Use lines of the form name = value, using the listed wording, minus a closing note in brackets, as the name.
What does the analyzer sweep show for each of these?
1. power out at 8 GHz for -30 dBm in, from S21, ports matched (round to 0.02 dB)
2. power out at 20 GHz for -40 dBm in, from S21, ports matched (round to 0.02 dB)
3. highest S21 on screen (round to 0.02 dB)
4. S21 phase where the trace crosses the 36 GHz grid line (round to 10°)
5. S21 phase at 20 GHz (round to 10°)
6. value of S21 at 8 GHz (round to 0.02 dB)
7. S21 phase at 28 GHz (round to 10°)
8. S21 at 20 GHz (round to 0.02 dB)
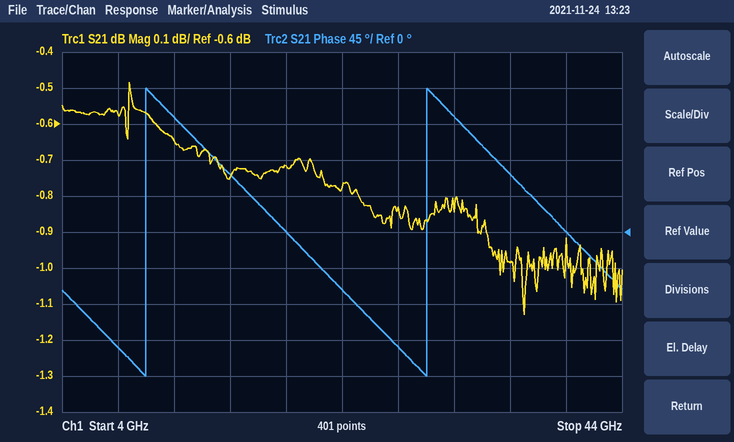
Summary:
power out at 8 GHz for -30 dBm in, from S21, ports matched = -30.58 dBm
power out at 20 GHz for -40 dBm in, from S21, ports matched = -40.72 dBm
highest S21 on screen = -0.48 dB
S21 phase where the trace crosses the 36 GHz grid line = 70°
S21 phase at 20 GHz = 0°
value of S21 at 8 GHz = -0.58 dB
S21 phase at 28 GHz = -140°
S21 at 20 GHz = -0.72 dB
